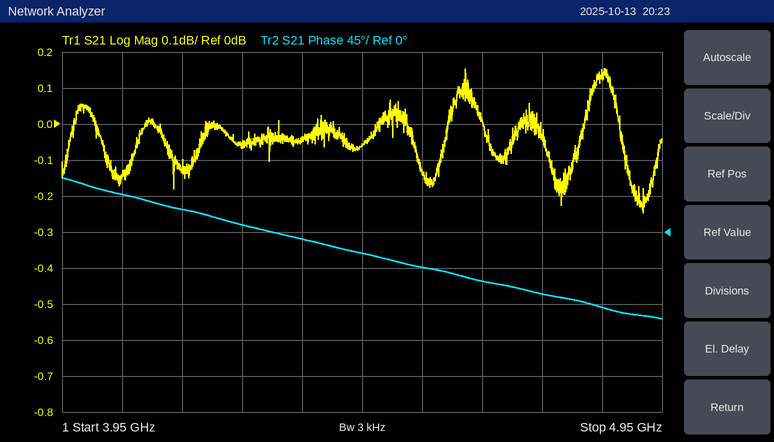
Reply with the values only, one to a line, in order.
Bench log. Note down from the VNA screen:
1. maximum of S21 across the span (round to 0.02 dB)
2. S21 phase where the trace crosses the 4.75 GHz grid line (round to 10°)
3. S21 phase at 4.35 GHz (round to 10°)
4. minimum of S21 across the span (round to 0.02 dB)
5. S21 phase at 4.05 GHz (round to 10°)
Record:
0.16 dB
-80°
-10°
-0.24 dB
50°
